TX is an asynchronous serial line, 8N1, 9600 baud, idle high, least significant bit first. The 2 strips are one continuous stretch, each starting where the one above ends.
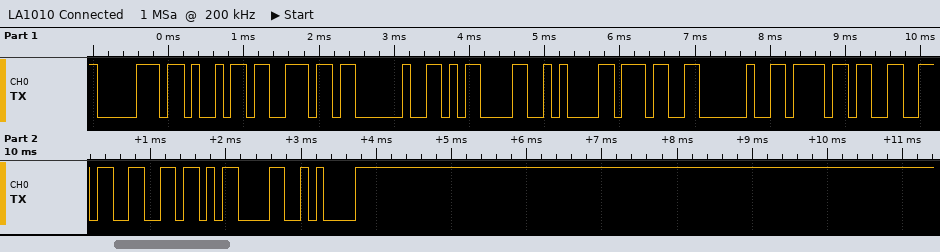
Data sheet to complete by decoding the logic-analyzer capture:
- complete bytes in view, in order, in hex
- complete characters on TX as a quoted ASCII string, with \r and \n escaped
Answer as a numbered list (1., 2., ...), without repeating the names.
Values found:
1. 0x70 0x69 0x6E 0x20 0x0D 0x0A 0x37 0x20 0x6F 0x66 0x66 0x0D 0x0A
2. "pin \r\n7 off\r\n"
